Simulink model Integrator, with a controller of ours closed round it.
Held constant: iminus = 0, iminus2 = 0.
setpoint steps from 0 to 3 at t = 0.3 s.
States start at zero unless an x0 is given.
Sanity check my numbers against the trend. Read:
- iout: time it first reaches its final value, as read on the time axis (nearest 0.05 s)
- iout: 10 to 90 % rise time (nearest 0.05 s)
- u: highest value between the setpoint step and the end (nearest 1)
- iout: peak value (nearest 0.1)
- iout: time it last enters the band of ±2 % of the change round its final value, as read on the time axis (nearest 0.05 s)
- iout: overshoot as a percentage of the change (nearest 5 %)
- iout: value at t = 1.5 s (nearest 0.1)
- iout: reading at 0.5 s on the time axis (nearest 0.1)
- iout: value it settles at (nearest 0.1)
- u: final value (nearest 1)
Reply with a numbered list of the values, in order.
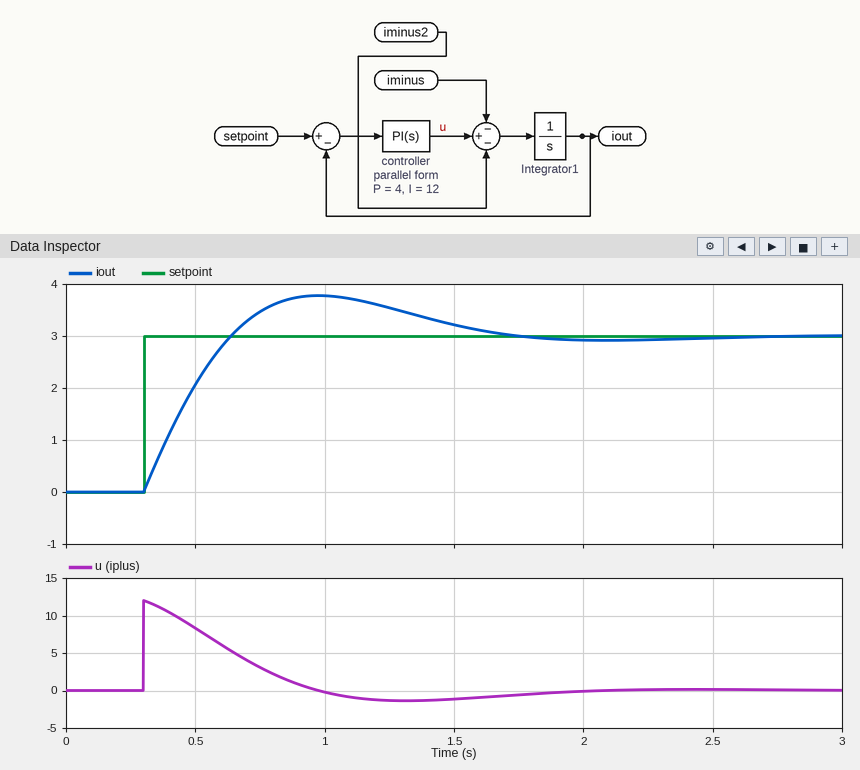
1. 0.65 s
2. 0.25 s
3. 12
4. 3.8
5. 2.35 s
6. 25 %
7. 3.2
8. 2.1
9. 3.0
10. 0
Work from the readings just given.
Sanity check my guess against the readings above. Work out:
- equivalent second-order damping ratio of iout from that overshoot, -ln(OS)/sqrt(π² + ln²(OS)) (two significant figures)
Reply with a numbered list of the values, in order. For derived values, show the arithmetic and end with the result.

1. ln(0.25) = -1.386; 1.386 / sqrt(9.870 + 1.922) = 0.40
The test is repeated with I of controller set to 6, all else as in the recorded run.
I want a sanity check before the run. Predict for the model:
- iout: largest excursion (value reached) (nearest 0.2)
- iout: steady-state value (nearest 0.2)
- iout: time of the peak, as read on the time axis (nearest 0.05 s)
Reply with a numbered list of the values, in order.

1. 3.6
2. 3.0
3. 1.15 s
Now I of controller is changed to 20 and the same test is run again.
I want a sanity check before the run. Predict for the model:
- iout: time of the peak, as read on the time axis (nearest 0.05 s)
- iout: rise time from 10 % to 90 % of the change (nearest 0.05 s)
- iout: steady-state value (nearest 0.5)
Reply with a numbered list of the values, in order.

1. 0.85 s
2. 0.20 s
3. 3.0
